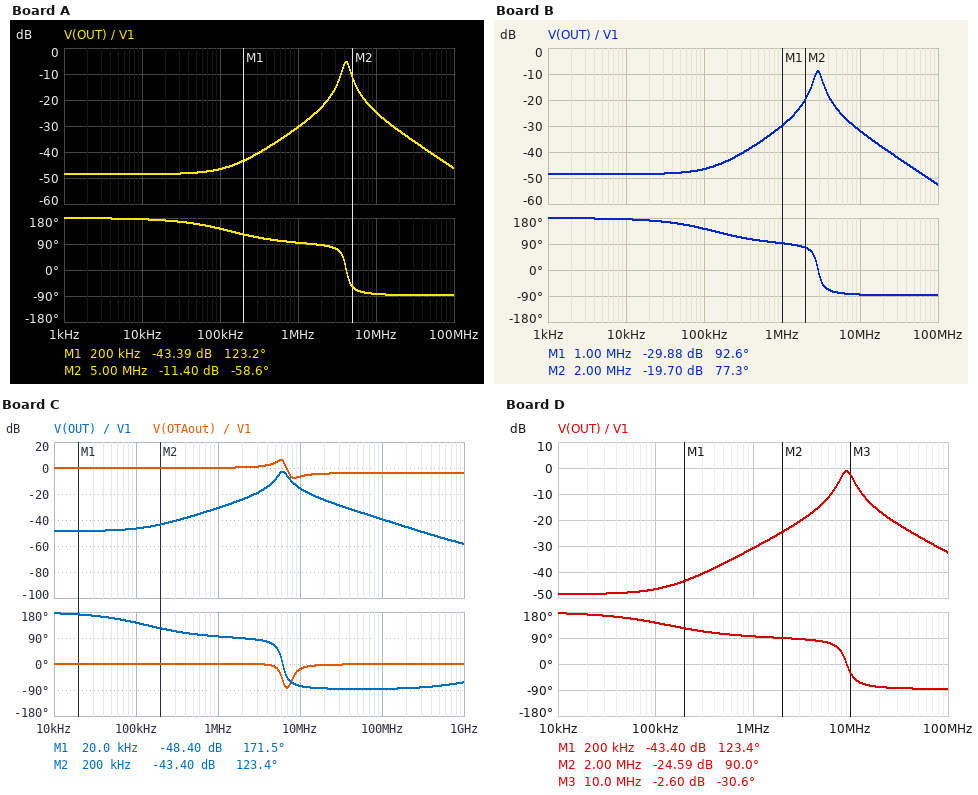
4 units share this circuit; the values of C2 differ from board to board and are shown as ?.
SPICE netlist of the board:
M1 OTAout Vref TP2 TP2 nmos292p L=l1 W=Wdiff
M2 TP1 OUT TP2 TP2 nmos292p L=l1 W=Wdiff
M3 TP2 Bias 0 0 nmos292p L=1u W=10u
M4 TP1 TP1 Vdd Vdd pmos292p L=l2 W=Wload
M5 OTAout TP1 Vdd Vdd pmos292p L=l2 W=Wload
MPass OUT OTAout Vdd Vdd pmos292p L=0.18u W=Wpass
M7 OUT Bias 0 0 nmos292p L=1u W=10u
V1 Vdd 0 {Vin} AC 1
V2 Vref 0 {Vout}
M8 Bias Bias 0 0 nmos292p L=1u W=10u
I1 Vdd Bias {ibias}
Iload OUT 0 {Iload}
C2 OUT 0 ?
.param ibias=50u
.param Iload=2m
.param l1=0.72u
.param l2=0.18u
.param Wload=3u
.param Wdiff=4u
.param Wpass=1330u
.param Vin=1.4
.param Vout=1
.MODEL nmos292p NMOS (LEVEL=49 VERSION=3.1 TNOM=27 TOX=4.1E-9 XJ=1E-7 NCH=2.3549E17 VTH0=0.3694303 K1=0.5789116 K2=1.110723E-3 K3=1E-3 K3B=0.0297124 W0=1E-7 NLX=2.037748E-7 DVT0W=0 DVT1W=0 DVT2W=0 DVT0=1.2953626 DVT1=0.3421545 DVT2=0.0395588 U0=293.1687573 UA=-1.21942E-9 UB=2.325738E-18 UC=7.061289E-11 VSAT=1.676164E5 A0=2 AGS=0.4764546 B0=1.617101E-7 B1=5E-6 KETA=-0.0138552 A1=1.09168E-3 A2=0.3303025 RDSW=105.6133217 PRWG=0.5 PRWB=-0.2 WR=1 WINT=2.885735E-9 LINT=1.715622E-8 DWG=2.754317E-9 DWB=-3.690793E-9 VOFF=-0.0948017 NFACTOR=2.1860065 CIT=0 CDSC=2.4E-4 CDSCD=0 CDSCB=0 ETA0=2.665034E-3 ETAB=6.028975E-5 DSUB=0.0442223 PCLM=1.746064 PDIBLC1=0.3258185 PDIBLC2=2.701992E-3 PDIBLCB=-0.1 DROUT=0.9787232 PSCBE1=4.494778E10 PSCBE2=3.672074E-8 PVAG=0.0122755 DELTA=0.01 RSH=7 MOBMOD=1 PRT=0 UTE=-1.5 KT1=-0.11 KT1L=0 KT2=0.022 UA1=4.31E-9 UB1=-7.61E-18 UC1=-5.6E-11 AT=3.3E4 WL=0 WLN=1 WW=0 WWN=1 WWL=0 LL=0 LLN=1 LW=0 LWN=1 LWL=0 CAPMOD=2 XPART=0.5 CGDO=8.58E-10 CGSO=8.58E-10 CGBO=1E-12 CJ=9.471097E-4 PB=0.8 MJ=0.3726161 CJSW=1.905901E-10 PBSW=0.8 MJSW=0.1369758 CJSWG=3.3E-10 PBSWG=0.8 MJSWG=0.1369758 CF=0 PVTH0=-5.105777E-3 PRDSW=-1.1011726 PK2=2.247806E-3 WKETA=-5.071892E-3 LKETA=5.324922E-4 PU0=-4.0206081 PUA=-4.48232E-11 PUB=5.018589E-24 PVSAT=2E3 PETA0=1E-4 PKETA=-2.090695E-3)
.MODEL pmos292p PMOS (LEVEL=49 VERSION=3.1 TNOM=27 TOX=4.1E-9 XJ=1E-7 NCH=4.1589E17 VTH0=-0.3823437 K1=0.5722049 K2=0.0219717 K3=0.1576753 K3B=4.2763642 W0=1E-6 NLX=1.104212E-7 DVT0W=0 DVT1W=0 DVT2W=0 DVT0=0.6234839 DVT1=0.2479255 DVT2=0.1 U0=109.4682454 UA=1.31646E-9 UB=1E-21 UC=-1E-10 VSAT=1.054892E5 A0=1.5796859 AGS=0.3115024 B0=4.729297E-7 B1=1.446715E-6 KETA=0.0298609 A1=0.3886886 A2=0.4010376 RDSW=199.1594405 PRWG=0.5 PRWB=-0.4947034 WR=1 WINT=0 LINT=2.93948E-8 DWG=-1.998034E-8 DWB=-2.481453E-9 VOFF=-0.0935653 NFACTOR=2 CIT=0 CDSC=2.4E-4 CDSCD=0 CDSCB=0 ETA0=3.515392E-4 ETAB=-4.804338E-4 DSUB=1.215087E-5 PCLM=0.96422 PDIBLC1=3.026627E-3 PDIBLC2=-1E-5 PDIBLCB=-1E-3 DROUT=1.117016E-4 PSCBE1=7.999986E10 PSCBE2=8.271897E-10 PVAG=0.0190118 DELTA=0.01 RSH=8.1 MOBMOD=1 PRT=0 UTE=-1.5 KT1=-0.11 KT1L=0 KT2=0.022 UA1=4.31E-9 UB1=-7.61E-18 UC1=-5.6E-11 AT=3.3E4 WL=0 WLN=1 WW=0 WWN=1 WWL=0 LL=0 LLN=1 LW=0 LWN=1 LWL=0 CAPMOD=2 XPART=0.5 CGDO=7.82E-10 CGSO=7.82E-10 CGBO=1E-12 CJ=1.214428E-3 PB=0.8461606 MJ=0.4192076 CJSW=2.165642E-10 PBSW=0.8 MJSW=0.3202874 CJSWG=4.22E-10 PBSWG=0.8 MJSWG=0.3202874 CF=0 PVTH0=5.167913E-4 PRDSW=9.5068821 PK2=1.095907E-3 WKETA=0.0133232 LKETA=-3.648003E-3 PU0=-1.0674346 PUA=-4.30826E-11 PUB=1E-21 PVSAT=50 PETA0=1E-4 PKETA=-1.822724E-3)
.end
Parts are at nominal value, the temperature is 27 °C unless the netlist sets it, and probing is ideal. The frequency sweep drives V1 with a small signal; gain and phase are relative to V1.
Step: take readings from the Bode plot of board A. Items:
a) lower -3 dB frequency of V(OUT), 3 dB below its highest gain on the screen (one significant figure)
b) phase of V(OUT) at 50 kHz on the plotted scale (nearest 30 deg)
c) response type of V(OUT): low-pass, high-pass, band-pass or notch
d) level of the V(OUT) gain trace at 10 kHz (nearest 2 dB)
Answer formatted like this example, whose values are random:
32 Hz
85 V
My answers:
4 MHz
150 deg
band-pass
-48 dB
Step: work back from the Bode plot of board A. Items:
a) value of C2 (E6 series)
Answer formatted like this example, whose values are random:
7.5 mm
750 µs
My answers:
3.3 nF
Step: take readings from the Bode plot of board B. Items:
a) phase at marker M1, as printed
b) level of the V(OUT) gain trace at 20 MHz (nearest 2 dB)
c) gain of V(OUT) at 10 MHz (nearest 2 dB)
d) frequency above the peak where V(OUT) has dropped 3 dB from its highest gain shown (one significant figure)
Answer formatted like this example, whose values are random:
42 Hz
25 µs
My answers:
92.6 deg
-38 dB
-32 dB
3 MHz
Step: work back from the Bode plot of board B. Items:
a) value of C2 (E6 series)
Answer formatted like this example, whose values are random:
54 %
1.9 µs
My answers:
6.8 nF
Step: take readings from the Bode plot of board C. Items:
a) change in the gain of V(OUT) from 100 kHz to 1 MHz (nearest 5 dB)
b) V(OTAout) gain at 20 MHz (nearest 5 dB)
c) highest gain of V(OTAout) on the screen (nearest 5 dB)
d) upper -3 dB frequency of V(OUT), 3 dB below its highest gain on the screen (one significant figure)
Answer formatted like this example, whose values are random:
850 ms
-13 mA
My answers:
15 dB
-5 dB
5 dB
7 MHz
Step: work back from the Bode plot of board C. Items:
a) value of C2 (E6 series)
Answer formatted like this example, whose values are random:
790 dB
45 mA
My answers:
1.5 nF
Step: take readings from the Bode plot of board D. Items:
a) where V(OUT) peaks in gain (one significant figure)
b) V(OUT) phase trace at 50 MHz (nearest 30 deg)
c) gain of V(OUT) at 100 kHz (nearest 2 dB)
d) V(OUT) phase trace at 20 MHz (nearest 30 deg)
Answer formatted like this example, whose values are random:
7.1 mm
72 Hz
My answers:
9 MHz
-90 deg
-46 dB
-90 deg
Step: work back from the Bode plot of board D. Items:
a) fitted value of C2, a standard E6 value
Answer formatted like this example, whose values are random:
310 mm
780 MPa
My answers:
680 pF
